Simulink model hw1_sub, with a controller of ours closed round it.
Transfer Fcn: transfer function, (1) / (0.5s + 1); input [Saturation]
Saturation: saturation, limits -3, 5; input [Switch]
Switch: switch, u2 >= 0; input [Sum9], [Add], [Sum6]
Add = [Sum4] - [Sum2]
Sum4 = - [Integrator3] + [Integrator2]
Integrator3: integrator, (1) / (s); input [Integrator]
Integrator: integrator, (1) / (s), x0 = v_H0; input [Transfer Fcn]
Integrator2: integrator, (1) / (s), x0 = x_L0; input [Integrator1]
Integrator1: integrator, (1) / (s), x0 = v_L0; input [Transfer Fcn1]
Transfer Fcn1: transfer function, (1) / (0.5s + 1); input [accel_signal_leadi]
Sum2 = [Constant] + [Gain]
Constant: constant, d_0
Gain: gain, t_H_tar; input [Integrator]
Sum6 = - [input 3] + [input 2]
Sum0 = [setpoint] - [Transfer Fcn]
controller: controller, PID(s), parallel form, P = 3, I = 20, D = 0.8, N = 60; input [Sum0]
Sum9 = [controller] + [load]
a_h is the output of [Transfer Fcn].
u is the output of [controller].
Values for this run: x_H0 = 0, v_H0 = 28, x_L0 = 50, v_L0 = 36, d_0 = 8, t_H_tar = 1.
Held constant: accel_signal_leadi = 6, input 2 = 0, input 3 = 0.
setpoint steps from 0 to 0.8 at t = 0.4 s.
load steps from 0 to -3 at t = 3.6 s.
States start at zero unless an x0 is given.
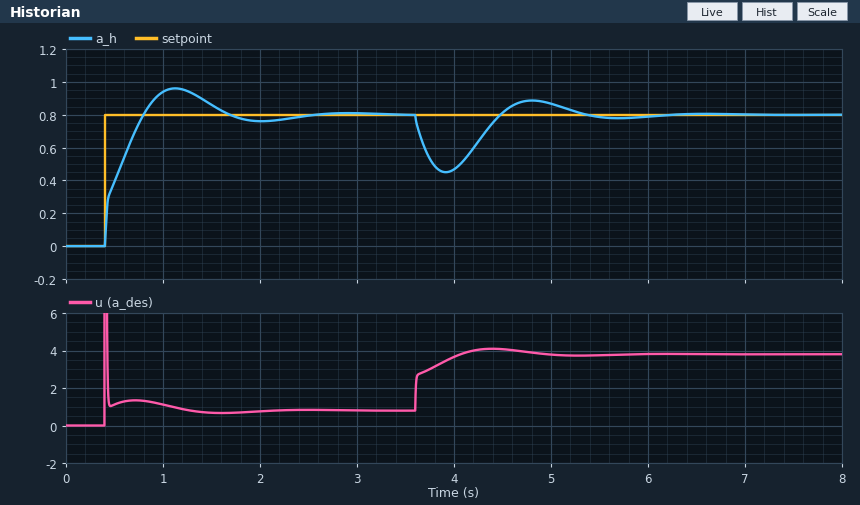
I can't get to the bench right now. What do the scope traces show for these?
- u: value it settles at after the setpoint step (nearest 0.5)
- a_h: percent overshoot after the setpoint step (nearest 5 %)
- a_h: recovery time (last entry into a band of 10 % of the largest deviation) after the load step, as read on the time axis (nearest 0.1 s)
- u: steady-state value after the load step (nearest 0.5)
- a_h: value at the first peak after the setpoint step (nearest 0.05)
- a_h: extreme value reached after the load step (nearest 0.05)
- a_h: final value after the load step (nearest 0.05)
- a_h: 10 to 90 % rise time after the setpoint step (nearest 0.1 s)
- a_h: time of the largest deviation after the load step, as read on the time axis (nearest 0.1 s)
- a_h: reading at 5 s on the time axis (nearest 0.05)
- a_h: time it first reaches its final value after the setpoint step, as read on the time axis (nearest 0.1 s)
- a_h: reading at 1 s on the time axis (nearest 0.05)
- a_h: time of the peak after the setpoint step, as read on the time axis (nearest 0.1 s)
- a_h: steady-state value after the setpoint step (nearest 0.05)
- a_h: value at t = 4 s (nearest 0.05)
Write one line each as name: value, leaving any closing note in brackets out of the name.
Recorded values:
u: value it settles at after the setpoint step: 1.0
a_h: percent overshoot after the setpoint step: 20 %
a_h: recovery time (last entry into a band of 10 % of the largest deviation) after the load step, as read on the time axis: 5.2 s
u: steady-state value after the load step: 4.0
a_h: value at the first peak after the setpoint step: 0.95
a_h: extreme value reached after the load step: 0.45
a_h: final value after the load step: 0.80
a_h: 10 to 90 % rise time after the setpoint step: 0.3 s
a_h: time of the largest deviation after the load step, as read on the time axis: 3.9 s
a_h: reading at 5 s on the time axis: 0.85
a_h: time it first reaches its final value after the setpoint step, as read on the time axis: 0.8 s
a_h: reading at 1 s on the time axis: 0.95
a_h: time of the peak after the setpoint step, as read on the time axis: 1.1 s
a_h: steady-state value after the setpoint step: 0.80
a_h: value at t = 4 s: 0.45
